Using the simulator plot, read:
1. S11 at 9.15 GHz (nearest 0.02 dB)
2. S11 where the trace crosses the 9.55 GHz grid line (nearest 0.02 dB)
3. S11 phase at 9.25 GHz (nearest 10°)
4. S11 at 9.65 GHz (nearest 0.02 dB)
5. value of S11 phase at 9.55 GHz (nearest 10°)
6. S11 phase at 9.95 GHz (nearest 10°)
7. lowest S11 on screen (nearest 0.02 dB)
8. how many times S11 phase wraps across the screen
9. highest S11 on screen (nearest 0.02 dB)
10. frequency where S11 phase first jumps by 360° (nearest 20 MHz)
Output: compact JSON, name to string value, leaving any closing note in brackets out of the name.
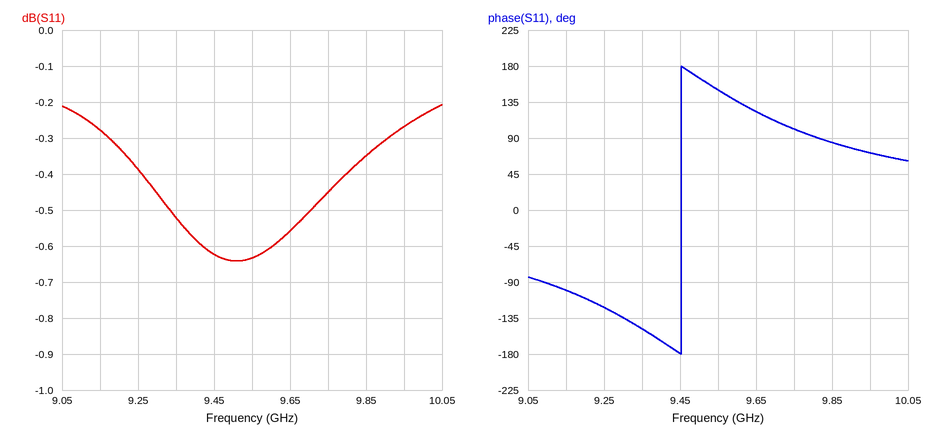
{"S11 at 9.15 GHz": "-0.28 dB", "S11 where the trace crosses the 9.55 GHz grid line": "-0.64 dB", "S11 phase at 9.25 GHz": "-120°", "S11 at 9.65 GHz": "-0.56 dB", "value of S11 phase at 9.55 GHz": "150°", "S11 phase at 9.95 GHz": "70°", "lowest S11 on screen": "-0.64 dB", "how many times S11 phase wraps across the screen": "1", "highest S11 on screen": "-0.20 dB", "frequency where S11 phase first jumps by 360°": "9.46 GHz"}
